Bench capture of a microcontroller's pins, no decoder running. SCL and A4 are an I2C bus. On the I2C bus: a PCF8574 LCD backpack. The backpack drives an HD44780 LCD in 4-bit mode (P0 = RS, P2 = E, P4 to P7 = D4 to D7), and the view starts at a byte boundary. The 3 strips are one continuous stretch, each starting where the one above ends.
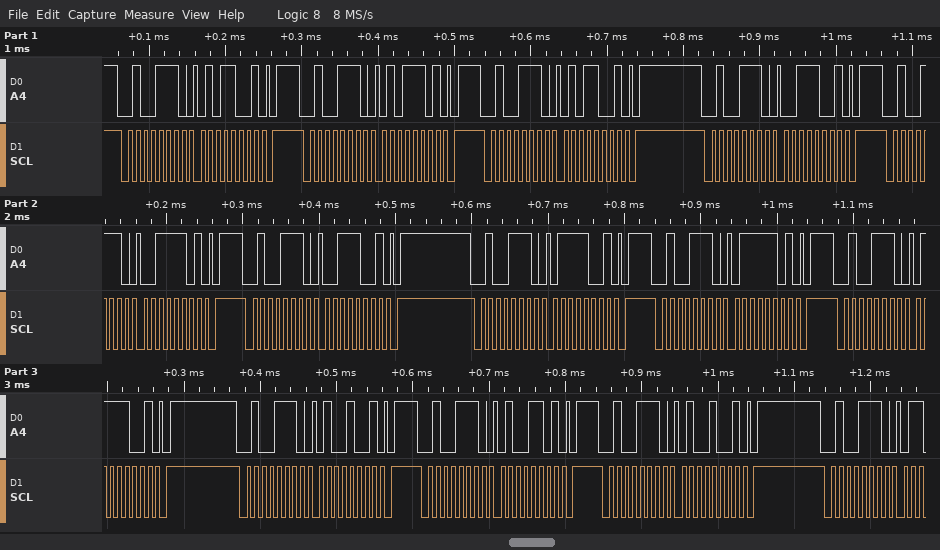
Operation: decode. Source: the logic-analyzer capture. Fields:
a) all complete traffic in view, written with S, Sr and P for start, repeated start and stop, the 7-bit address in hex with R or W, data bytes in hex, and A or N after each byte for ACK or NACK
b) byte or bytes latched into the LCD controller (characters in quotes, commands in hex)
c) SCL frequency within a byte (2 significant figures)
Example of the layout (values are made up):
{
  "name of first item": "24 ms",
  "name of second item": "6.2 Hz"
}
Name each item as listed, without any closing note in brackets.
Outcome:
{
  "all complete traffic in view, written with S, Sr and P for start, repeated start and stop, the 7-bit address in hex with R or W, data bytes in hex, and A or N after each byte for ACK or NACK": "S 27W A 59 A P S 27W A 5D A P S 27W A 59 A P S 27W A 39 A P S 27W A 3D A P S 27W A 39 A P S 27W A 79 A P S 27W A 7D A P S 27W A 79 A P S 27W A 49 A P S 27W A 4D A P S 27W A 49 A P S 27W A",
  "byte or bytes latched into the LCD controller": "'S' 't'",
  "SCL frequency within a byte": "100 kHz"
}
